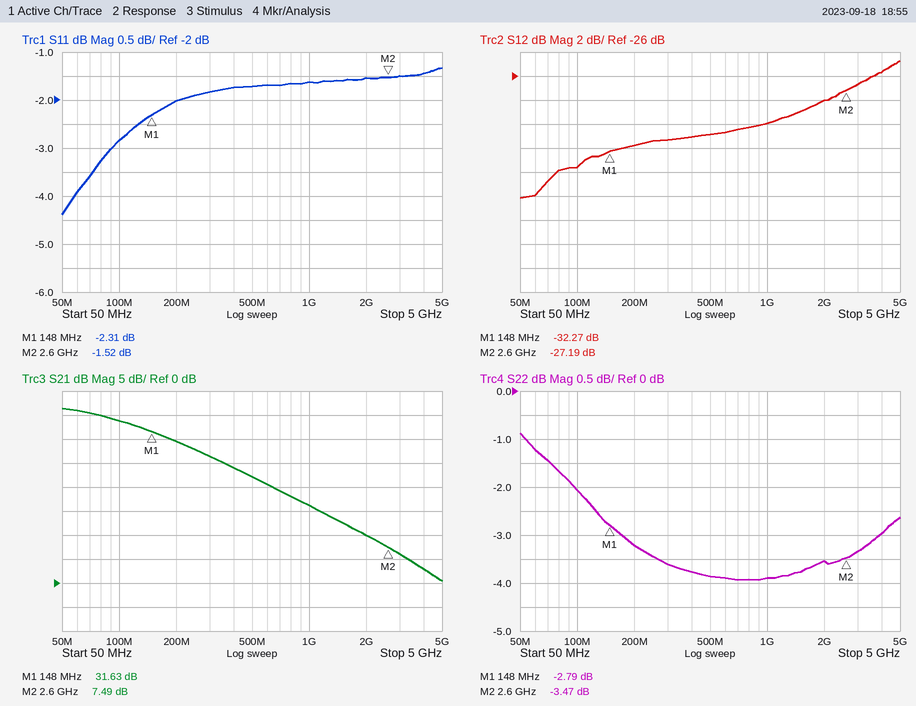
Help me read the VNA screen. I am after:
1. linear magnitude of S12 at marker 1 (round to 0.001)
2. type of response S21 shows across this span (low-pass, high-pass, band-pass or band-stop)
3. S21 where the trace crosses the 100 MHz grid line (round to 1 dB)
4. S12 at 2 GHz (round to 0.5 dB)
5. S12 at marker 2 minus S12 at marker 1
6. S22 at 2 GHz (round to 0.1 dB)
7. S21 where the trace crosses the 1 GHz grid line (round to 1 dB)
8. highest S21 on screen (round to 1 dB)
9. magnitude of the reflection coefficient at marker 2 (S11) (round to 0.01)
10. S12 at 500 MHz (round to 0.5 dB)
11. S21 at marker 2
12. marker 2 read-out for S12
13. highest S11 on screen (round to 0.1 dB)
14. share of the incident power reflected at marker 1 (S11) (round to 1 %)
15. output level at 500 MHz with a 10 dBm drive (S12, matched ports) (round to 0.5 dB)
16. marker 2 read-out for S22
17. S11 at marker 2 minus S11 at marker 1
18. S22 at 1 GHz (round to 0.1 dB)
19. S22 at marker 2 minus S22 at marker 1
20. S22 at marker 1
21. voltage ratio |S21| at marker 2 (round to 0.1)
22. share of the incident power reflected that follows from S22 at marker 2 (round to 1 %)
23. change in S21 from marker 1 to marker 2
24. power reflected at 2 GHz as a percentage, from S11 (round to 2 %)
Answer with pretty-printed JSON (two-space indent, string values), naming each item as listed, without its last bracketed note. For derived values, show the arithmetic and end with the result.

{
  "linear magnitude of S12 at marker 1": "10^(-32.27/20) ≈ 0.024",
  "type of response S21 shows across this span": "low-pass",
  "S21 where the trace crosses the 100 MHz grid line": "34 dB",
  "S12 at 2 GHz": "-28.0 dB",
  "S12 at marker 2 minus S12 at marker 1": "-27.19 − (-32.27) = 5.08 dB",
  "S22 at 2 GHz": "-3.5 dB",
  "S21 where the trace crosses the 1 GHz grid line": "16 dB",
  "highest S21 on screen": "36 dB",
  "magnitude of the reflection coefficient at marker 2 (S11)": "10^(-1.52/20) ≈ 0.84",
  "S12 at 500 MHz": "-31.0 dB",
  "S21 at marker 2": "7.49 dB",
  "marker 2 read-out for S12": "-27.19 dB",
  "highest S11 on screen": "-1.3 dB",
  "share of the incident power reflected at marker 1 (S11)": "10^(-2.31/10) ≈ 59 %",
  "output level at 500 MHz with a 10 dBm drive (S12, matched ports)": "10 dBm + (-31.0 dB) = -21.0 dBm",
  "marker 2 read-out for S22": "-3.47 dB",
  "S11 at marker 2 minus S11 at marker 1": "-1.52 − (-2.31) = 0.79 dB",
  "S22 at 1 GHz": "-3.9 dB",
  "S22 at marker 2 minus S22 at marker 1": "-3.47 − (-2.79) = -0.68 dB",
  "S22 at marker 1": "-2.79 dB",
  "voltage ratio |S21| at marker 2": "10^(7.49/20) ≈ 2.4",
  "share of the incident power reflected that follows from S22 at marker 2": "10^(-3.47/10) ≈ 45 %",
  "change in S21 from marker 1 to marker 2": "7.49 − (31.63) = -24.14 dB",
  "power reflected at 2 GHz as a percentage, from S11": "10^(-1.5/10) ≈ 70.8 %, so 70 % to the nearest 2 %"
}
